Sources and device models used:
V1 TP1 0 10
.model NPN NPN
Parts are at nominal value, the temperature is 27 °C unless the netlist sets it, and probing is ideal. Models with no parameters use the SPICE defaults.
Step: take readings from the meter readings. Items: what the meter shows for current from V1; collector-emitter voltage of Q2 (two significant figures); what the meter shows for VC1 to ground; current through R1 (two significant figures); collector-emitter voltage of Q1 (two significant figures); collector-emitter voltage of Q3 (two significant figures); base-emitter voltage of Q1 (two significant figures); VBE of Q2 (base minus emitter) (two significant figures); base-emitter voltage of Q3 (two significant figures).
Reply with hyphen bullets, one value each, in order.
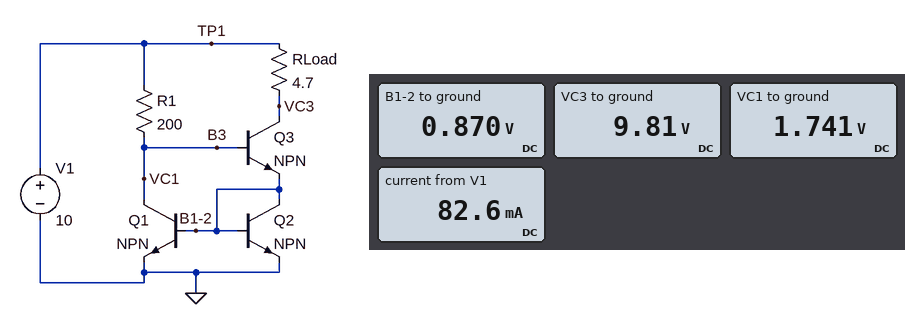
- 82.6 mA
- 870 mV
- 1.741 V
- 41 mA
- 1.7 V
- 8.9 V
- 870 mV
- 870 mV
- 870 mV
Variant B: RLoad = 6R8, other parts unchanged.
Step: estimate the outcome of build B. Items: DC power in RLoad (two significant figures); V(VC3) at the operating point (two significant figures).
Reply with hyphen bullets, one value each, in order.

- 12 mW
- 9.7 V
